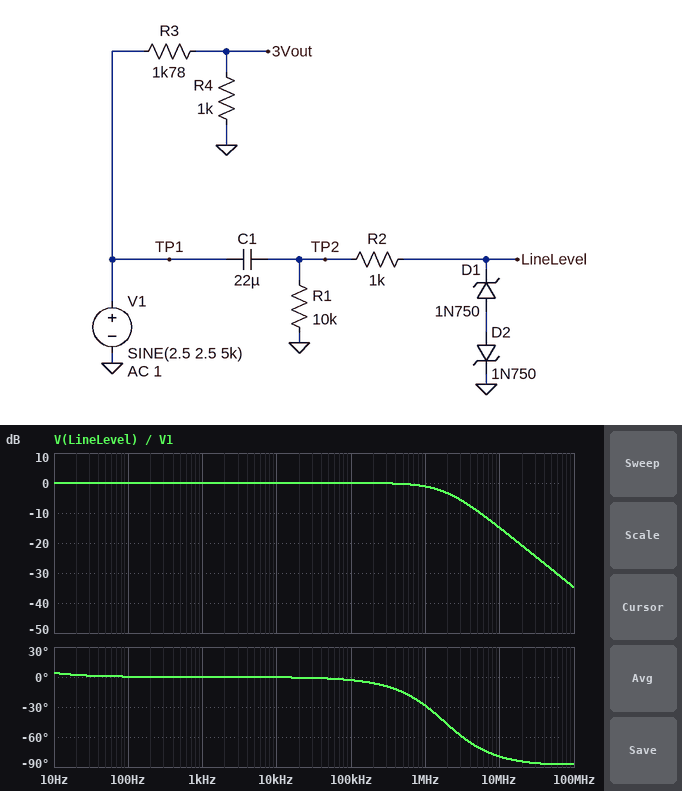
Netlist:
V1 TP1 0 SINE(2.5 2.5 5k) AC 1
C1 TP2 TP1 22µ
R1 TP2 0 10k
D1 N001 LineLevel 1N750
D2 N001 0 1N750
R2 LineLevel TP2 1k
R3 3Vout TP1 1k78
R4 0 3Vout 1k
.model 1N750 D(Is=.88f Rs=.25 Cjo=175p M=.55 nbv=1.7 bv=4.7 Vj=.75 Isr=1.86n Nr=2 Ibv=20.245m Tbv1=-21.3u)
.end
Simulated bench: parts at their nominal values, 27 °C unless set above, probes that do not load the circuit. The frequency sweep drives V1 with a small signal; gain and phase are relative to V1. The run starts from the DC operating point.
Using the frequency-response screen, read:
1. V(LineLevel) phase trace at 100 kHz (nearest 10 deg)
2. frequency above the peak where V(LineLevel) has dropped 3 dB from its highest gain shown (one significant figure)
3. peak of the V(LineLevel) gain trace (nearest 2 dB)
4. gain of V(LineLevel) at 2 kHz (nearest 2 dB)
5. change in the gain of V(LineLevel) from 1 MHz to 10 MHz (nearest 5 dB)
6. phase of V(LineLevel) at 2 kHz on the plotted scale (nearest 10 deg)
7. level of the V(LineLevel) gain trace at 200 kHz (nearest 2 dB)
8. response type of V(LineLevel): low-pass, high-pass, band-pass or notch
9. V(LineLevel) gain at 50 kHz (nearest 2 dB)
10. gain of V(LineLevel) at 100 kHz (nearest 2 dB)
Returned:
0 deg
2 MHz
0 dB
0 dB
-15 dB
0 deg
0 dB
low-pass
0 dB
0 dB
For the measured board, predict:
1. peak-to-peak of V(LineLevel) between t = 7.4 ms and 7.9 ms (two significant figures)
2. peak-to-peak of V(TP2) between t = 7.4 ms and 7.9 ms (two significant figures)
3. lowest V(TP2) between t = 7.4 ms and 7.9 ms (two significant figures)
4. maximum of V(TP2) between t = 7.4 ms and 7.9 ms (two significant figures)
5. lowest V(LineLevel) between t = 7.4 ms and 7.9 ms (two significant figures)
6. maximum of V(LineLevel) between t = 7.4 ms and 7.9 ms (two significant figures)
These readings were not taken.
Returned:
5.0 V
5.0 V
-2.5 V
2.5 V
-2.5 V
2.5 V
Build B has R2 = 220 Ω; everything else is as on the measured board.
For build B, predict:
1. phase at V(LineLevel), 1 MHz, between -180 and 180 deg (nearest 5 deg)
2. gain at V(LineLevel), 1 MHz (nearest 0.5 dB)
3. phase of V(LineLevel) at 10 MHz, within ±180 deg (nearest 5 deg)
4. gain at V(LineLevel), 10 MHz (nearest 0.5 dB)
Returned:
-5 deg
0 dB
-50 deg
-4.0 dB
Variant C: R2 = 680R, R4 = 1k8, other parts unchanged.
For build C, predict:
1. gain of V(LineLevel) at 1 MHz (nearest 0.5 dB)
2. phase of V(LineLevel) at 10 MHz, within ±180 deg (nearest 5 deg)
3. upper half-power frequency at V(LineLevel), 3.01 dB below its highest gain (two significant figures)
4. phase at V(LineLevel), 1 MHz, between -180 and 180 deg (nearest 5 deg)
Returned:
-0.5 dB
-75 deg
2.7 MHz
-20 deg
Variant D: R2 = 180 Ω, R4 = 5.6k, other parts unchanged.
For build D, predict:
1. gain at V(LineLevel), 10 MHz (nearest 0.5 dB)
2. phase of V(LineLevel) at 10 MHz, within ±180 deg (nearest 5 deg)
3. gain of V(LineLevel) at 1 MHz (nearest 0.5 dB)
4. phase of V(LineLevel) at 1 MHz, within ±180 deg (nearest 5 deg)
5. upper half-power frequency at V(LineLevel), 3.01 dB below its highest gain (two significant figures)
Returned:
-3.0 dB
-45 deg
0 dB
-5 deg
10 MHz
